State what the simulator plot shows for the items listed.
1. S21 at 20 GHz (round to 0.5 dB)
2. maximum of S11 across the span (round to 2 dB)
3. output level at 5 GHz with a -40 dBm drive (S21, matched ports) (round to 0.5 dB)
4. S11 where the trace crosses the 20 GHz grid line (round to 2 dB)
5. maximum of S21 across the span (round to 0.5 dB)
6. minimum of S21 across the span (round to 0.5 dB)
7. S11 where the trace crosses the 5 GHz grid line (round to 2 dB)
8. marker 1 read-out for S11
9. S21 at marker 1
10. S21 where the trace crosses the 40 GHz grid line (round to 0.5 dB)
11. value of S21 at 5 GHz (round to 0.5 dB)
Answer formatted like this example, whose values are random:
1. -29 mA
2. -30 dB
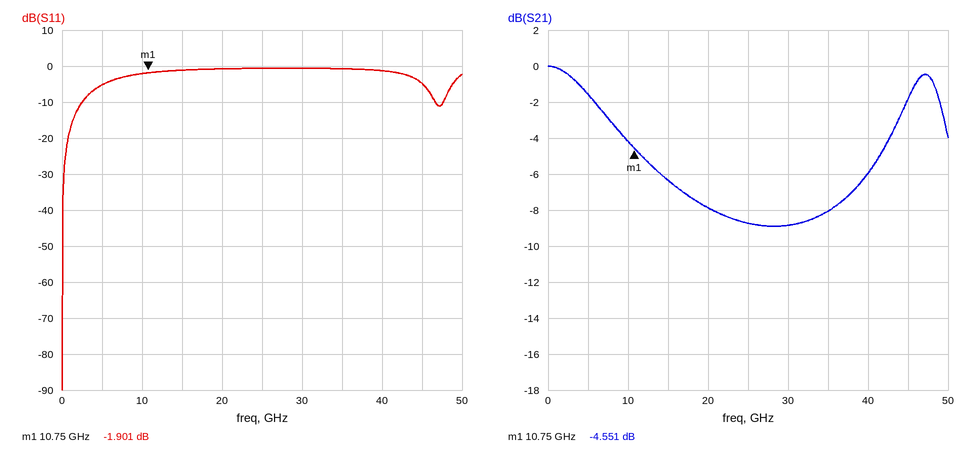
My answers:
1. -8.0 dB
2. 0 dB
3. -41.5 dBm
4. 0 dB
5. 0.0 dB
6. -9.0 dB
7. -6 dB
8. -1.901 dB
9. -4.551 dB
10. -6.0 dB
11. -1.5 dB
